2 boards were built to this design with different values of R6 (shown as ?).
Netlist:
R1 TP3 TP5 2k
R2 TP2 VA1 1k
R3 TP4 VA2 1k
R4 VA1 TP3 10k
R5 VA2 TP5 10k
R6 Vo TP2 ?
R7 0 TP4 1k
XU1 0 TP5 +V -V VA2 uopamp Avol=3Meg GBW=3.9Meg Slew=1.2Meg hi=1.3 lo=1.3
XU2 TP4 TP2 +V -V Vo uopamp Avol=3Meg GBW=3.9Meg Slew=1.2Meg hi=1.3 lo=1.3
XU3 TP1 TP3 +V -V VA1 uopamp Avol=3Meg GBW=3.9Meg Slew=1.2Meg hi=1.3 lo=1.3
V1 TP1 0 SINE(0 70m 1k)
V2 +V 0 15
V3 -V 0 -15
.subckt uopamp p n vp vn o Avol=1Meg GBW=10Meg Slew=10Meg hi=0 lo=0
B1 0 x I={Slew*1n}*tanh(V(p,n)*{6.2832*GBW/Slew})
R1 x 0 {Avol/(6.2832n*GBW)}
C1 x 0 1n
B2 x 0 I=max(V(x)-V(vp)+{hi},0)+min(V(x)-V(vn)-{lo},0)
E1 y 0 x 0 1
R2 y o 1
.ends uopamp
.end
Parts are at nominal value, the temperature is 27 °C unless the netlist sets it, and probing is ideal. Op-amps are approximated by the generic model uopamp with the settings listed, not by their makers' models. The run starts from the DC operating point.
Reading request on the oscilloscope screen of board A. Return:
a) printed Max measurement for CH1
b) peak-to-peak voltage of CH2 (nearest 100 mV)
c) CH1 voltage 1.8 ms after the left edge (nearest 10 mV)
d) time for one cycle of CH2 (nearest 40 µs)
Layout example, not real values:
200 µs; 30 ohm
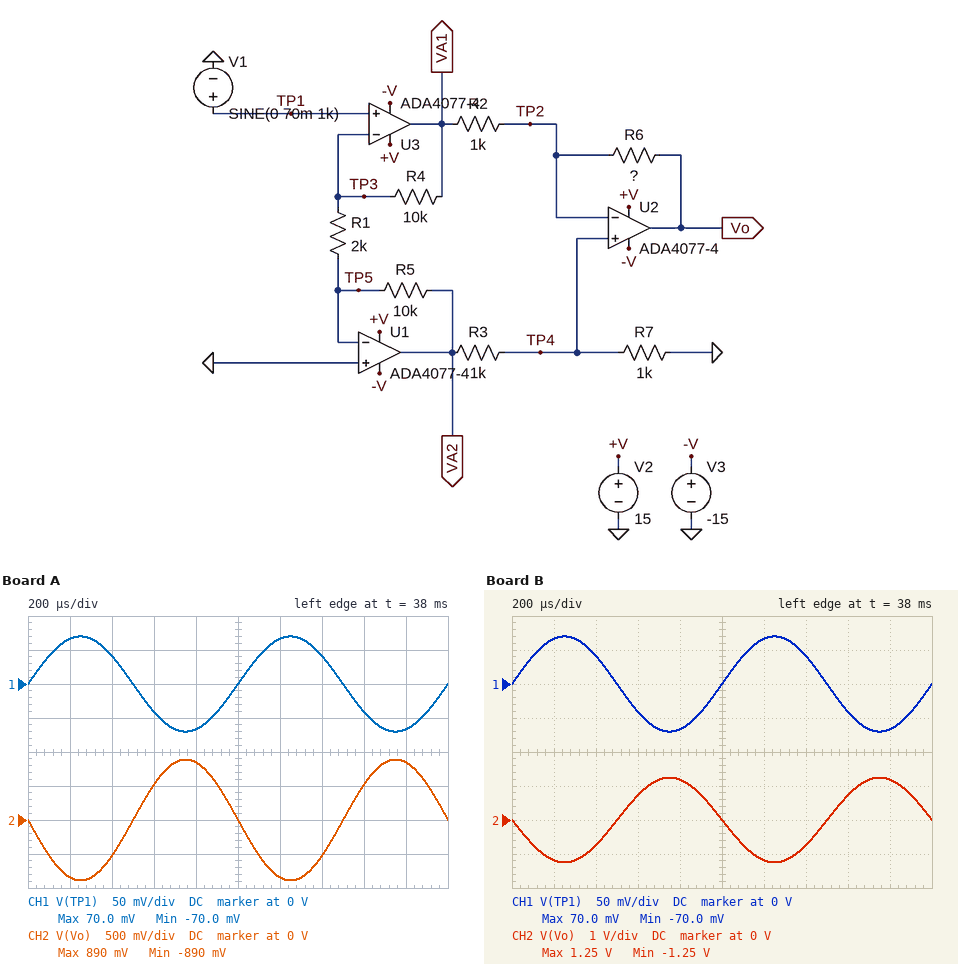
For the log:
70.0 mV; 1.8 V; -70 mV; 1.00 ms
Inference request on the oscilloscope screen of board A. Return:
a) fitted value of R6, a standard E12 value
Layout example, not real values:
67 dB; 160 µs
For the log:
1.2 kΩ
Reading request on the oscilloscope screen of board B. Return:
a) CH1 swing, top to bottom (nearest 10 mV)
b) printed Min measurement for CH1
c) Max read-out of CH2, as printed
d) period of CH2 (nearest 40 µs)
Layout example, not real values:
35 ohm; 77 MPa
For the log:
140 mV; -70.0 mV; 1.25 V; 1.00 ms
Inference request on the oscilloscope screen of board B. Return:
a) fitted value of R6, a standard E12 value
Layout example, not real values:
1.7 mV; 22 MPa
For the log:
1.8 kΩ
